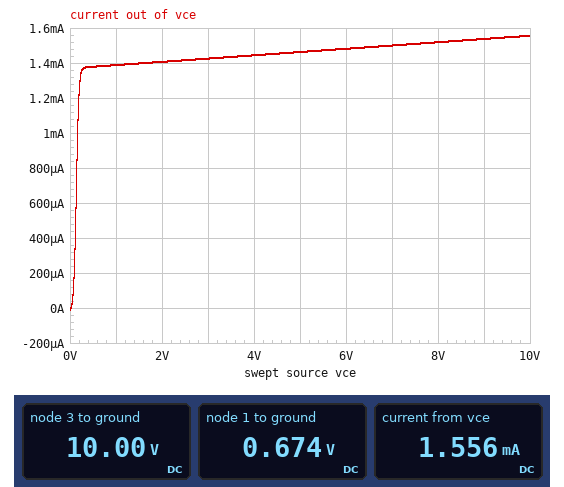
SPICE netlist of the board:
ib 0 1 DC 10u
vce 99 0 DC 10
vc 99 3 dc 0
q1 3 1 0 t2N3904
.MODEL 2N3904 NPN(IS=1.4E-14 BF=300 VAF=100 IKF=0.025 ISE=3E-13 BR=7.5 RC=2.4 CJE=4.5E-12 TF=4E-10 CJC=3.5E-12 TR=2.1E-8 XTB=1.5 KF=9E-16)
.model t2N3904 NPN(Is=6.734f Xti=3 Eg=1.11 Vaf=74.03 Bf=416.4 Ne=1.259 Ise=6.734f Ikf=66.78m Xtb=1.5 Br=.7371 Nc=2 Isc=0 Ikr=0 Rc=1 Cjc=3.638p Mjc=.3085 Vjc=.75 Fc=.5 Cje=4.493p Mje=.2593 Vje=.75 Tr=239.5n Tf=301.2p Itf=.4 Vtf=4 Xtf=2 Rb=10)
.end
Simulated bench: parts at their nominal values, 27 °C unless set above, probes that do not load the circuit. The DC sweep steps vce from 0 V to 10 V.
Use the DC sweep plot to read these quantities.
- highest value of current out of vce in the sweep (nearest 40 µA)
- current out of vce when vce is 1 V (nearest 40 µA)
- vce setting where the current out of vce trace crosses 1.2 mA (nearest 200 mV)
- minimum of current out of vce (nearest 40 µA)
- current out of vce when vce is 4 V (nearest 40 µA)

1.56 mA
1.40 mA
200 mV
0 A
1.44 mA
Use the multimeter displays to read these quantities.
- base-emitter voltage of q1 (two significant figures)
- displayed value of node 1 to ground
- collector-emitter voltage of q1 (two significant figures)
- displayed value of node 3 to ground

670 mV
0.674 V
10 V
10.00 V
